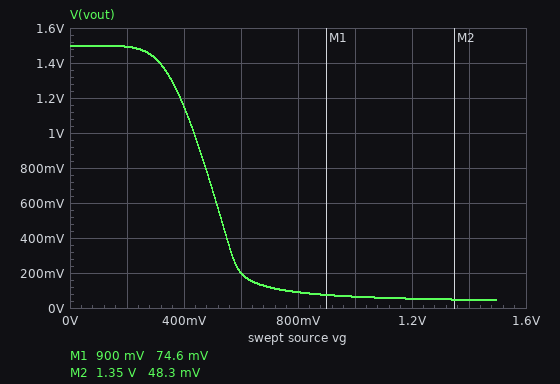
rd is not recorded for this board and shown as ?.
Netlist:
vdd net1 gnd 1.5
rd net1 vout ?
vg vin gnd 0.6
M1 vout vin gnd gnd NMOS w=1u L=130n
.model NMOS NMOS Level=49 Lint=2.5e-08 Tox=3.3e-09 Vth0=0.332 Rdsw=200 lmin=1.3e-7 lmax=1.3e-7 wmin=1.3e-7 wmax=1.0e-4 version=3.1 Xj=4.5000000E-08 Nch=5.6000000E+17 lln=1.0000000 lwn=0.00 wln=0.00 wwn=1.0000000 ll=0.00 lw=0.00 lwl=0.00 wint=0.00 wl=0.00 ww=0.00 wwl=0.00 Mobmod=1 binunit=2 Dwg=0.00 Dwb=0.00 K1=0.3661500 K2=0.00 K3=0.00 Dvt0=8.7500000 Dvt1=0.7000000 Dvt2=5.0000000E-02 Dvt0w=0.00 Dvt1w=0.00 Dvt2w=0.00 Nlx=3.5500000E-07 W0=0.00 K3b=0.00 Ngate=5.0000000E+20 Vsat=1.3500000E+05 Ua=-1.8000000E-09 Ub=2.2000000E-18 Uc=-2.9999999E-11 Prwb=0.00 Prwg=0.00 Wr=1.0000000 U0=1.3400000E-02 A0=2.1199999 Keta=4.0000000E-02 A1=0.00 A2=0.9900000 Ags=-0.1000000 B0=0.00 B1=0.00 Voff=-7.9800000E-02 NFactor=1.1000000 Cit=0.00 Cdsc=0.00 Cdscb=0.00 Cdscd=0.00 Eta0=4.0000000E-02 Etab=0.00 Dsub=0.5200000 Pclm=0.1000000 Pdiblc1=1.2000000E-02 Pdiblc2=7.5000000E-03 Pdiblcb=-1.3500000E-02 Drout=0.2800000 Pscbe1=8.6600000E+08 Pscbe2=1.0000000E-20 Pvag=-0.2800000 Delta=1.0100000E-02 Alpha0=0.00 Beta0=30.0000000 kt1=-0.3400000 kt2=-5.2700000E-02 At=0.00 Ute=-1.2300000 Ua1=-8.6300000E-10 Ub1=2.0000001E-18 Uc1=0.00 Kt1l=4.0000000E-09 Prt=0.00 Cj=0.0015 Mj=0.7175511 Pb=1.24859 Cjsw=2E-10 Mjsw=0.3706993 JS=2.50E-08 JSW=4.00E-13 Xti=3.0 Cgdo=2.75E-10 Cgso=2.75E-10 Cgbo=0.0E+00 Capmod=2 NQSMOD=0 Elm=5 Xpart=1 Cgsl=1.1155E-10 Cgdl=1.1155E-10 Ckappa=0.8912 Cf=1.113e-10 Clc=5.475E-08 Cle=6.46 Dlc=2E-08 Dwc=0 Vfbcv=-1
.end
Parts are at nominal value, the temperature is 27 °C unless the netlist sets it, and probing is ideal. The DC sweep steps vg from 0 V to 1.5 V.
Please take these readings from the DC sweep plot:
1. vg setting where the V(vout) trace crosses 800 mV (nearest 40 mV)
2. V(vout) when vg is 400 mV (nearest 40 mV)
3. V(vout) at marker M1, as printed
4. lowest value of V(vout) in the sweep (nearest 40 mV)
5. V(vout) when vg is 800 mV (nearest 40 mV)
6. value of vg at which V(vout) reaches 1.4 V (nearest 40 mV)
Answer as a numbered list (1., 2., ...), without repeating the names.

1. 480 mV
2. 1.16 V
3. 74.6 mV
4. 40 mV
5. 80 mV
6. 320 mV
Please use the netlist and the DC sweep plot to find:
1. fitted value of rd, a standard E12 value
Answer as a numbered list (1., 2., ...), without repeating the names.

1. 18 kΩ
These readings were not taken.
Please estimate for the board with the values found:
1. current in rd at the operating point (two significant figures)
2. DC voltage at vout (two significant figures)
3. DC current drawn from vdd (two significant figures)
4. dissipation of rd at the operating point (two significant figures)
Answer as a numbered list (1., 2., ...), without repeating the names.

1. 72 µA
2. 200 mV
3. 72 µA
4. 94 µW
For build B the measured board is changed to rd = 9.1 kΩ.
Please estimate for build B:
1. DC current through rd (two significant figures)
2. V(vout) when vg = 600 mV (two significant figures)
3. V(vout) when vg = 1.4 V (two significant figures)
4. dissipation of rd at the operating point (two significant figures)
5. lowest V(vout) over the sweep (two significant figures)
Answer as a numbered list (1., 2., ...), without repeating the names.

1. 90 µA
2. 680 mV
3. 94 mV
4. 74 µW
5. 90 mV
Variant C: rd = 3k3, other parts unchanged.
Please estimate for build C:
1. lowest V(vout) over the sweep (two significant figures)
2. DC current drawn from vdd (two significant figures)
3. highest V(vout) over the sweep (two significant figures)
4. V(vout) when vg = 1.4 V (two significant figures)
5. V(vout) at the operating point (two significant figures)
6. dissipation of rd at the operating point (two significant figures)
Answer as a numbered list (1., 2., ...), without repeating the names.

1. 250 mV
2. 100 µA
3. 1.5 V
4. 270 mV
5. 1.2 V
6. 34 µW
